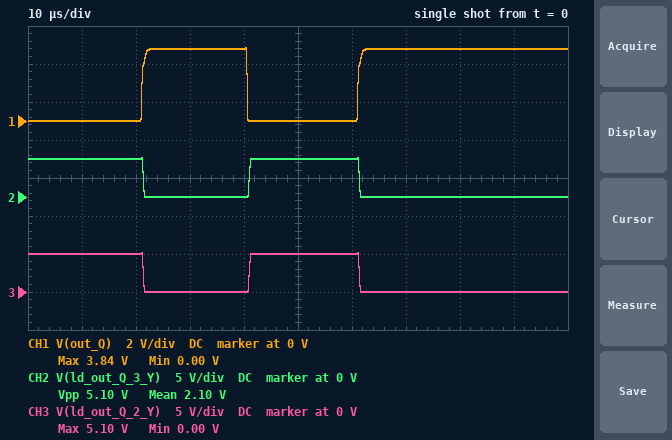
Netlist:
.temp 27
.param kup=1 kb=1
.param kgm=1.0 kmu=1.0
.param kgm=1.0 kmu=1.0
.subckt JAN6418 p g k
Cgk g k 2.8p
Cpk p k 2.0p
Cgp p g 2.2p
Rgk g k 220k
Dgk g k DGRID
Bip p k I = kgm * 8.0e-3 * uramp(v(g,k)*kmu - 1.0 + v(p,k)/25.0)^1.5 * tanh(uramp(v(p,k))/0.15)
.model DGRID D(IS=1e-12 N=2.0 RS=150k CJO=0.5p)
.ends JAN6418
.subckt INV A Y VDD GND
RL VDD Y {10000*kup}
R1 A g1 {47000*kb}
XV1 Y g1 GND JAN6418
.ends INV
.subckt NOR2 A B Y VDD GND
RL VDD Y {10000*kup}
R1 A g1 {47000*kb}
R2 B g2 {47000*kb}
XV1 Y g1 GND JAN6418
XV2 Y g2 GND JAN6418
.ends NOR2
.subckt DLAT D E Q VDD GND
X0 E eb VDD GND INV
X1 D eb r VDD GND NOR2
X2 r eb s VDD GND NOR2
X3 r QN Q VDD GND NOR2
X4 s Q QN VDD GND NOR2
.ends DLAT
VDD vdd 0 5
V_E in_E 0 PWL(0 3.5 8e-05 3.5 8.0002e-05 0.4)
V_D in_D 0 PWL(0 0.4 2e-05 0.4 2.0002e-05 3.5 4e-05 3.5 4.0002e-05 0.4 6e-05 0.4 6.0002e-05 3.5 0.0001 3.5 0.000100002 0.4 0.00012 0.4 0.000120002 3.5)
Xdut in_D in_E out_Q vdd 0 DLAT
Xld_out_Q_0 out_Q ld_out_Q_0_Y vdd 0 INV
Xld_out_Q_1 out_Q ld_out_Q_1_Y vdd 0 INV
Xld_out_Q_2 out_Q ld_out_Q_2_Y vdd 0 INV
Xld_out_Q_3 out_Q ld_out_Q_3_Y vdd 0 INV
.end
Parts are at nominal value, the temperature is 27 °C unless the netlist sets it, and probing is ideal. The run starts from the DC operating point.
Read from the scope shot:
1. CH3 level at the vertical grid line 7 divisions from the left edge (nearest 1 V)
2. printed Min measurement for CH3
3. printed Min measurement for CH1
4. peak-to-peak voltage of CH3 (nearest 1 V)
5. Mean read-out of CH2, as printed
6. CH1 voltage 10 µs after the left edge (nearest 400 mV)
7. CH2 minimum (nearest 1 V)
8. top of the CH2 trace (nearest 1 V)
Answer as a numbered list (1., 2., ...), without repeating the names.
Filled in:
1. 0 V
2. 0.00 V
3. 0.00 V
4. 5 V
5. 2.10 V
6. 0 V
7. 0 V
8. 5 V
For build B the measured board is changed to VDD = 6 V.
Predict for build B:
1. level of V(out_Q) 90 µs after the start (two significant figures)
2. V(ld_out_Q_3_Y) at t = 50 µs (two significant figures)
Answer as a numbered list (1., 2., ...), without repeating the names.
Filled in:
1. 4.5 V
2. 6.0 V
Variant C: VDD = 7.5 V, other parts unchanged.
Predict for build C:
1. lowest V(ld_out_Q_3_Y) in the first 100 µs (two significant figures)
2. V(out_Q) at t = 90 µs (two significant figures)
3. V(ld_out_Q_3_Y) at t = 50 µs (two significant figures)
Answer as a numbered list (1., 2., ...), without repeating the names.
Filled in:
1. 2.9 mV
2. 5.6 V
3. 7.5 V
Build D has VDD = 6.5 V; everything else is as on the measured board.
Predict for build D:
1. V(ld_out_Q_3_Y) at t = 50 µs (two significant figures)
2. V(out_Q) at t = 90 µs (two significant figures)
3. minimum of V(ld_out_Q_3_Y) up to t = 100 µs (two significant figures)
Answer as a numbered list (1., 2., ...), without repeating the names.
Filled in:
1. 6.5 V
2. 4.9 V
3. 3.3 mV
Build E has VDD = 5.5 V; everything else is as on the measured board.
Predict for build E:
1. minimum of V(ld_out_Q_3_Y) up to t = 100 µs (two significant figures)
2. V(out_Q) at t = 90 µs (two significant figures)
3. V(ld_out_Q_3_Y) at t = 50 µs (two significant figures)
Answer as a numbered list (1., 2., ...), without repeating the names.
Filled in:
1. 3.9 mV
2. 4.2 V
3. 5.5 V
